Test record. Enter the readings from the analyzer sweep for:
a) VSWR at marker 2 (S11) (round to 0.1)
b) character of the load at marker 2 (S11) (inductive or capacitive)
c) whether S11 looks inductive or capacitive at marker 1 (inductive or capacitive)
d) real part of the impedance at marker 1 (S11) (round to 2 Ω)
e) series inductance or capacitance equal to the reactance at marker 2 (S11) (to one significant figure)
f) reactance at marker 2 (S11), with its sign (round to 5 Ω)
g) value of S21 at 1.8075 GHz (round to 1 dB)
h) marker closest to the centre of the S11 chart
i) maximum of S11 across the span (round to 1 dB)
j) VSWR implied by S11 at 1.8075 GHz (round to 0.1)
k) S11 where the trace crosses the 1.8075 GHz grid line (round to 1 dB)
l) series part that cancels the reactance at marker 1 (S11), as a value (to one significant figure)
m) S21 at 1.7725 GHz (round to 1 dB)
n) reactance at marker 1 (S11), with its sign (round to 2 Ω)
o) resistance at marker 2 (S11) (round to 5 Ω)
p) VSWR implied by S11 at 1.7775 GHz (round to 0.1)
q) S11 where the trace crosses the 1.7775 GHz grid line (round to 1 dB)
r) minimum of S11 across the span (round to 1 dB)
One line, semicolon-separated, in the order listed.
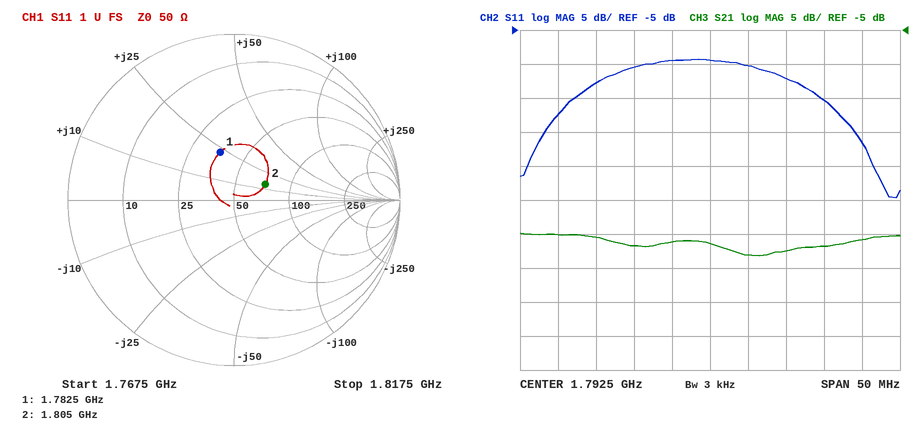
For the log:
1.5; inductive; inductive; 36 Ω; 1 nH; +15 Ω; -37 dB; marker 2; -9 dB; 1.4; -15 dB; 4 pF; -35 dB; +22 Ω; 70 Ω; 1.6; -13 dB; -30 dB
